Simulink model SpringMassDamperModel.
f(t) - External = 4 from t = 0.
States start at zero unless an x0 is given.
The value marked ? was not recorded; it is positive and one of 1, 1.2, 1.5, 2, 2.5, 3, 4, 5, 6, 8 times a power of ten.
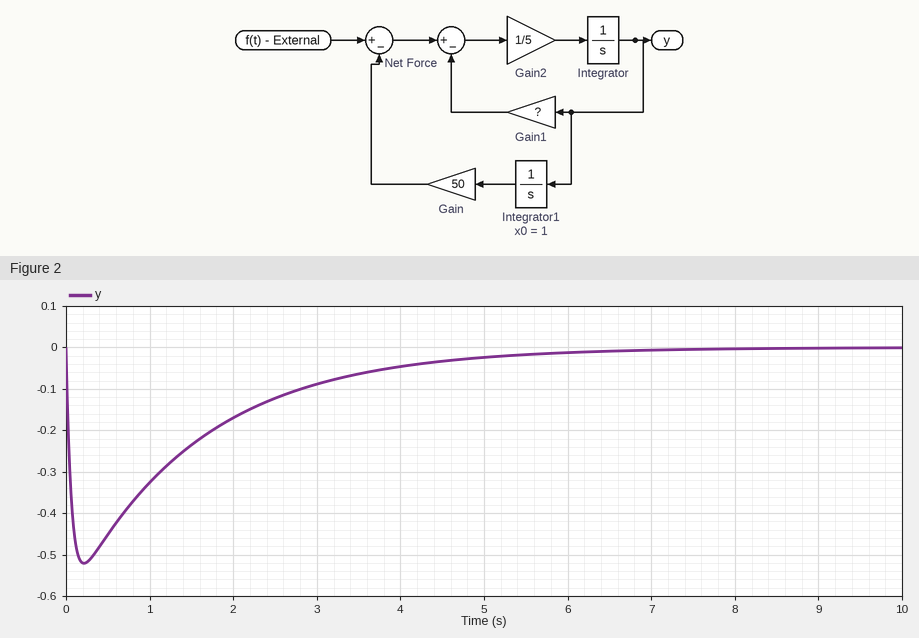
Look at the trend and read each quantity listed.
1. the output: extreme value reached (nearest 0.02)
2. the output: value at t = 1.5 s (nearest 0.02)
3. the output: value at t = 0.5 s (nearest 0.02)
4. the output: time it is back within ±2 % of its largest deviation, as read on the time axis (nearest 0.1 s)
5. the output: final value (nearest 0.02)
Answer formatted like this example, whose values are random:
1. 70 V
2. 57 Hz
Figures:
1. -0.52
2. -0.24
3. -0.46
4. 6.3 s
5. 0.00
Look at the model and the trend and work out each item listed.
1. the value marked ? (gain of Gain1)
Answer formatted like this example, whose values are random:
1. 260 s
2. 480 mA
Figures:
1. 80
